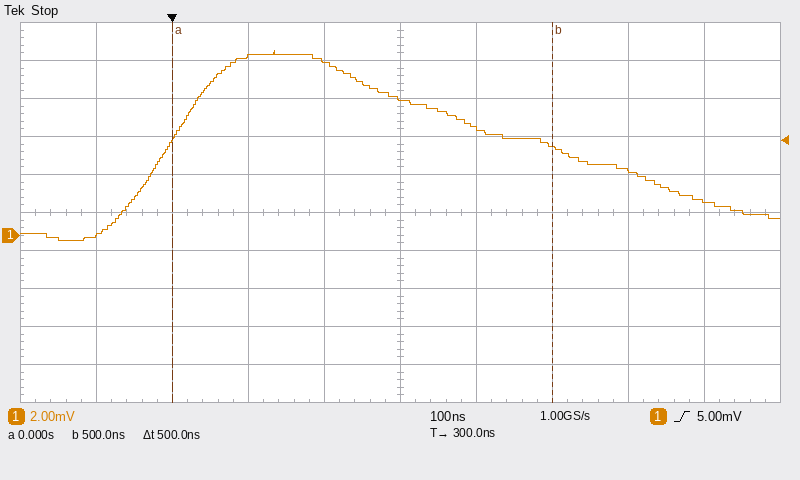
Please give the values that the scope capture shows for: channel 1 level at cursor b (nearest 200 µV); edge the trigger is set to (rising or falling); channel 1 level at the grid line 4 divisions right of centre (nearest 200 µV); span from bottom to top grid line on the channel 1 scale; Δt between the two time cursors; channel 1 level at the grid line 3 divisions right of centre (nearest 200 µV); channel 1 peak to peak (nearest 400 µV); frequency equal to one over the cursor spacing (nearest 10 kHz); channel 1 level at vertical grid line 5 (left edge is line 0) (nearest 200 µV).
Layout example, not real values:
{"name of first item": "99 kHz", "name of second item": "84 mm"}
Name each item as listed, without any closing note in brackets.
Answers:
{"channel 1 level at cursor b": "4.6 mV", "edge the trigger is set to": "rising", "channel 1 level at the grid line 4 divisions right of centre": "1.8 mV", "span from bottom to top grid line on the channel 1 scale": "20 mV", "Δt between the two time cursors": "500 ns", "channel 1 level at the grid line 3 divisions right of centre": "3.4 mV", "channel 1 peak to peak": "10.0 mV", "frequency equal to one over the cursor spacing": "2.00 MHz", "channel 1 level at vertical grid line 5 (left edge is line 0)": "7.2 mV"}
